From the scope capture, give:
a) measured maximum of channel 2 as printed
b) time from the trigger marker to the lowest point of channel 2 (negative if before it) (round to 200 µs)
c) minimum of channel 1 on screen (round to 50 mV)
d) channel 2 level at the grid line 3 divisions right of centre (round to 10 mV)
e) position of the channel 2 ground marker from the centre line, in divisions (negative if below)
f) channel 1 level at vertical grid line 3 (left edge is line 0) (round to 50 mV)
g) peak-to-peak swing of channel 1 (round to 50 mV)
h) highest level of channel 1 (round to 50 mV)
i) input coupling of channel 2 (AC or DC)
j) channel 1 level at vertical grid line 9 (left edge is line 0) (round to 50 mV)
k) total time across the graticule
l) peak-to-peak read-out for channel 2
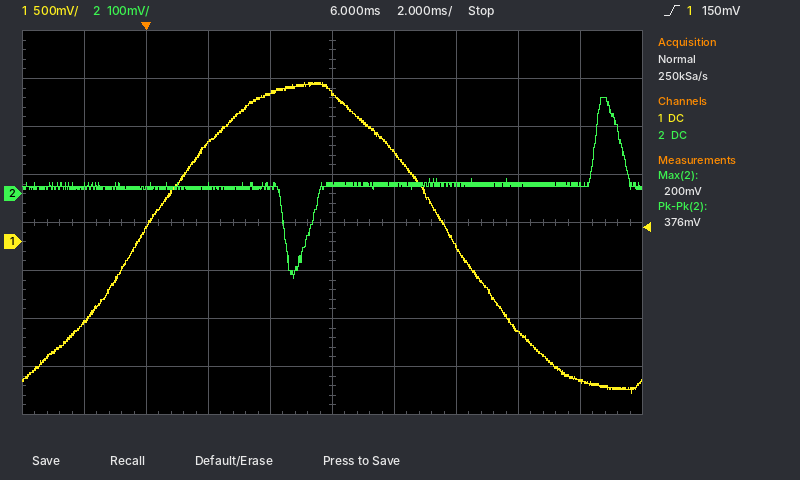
200 mV
+4.8 ms
-1.60 V
20 mV
+0.6 div
1.00 V
3.25 V
1.65 V
DC
-1.45 V
20 ms
376 mV
